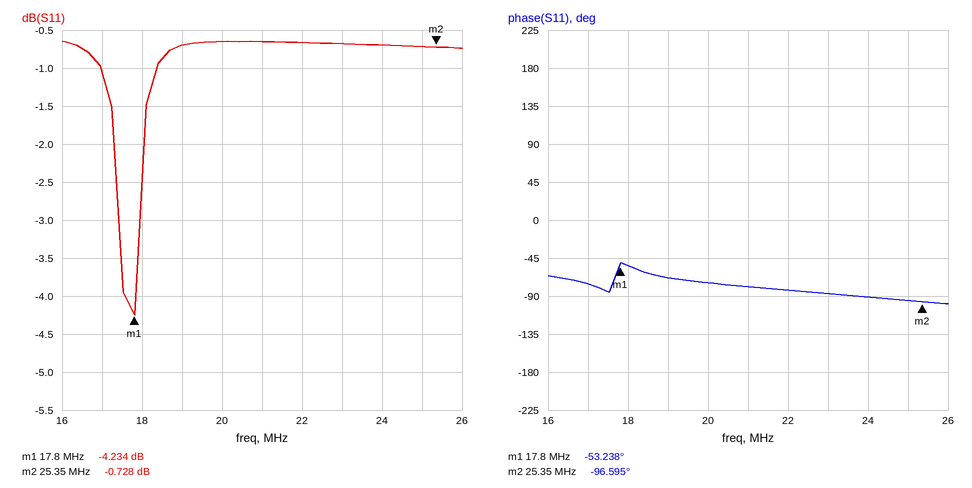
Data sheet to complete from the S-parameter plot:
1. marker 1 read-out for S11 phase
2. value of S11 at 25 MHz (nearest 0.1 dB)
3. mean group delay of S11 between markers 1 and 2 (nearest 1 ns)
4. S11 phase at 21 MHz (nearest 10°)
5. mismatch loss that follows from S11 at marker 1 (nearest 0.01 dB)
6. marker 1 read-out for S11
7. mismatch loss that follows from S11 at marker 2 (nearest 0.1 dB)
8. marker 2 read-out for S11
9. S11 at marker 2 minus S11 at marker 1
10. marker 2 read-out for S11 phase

-53.238°
-0.7 dB
16 ns
-80°
2.06 dB
-4.234 dB
8.1 dB
-0.728 dB
3.506 dB
-96.595°
